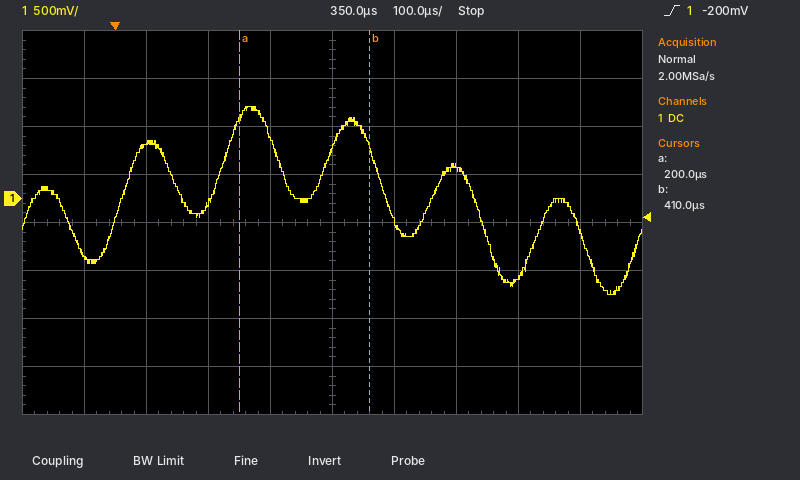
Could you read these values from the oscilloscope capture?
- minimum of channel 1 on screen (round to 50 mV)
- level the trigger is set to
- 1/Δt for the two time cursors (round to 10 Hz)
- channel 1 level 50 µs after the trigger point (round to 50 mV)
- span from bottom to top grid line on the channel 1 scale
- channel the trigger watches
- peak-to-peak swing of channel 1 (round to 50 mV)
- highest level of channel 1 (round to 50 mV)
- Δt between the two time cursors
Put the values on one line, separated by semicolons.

-1.00 V; -200 mV; 4.76 kHz; 550 mV; 4 V; channel 1; 1.95 V; 950 mV; 210 µs
